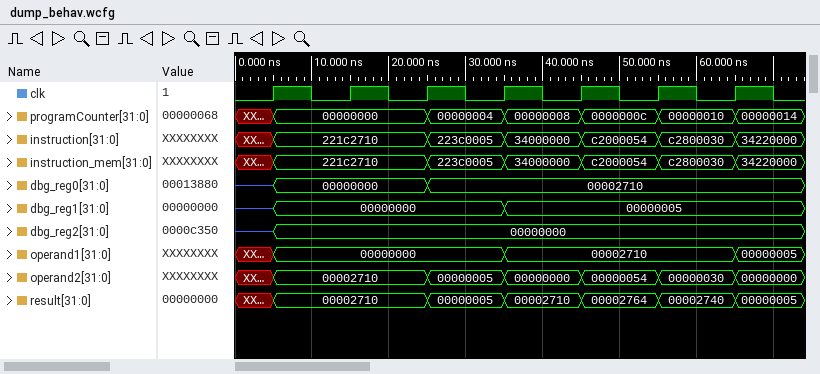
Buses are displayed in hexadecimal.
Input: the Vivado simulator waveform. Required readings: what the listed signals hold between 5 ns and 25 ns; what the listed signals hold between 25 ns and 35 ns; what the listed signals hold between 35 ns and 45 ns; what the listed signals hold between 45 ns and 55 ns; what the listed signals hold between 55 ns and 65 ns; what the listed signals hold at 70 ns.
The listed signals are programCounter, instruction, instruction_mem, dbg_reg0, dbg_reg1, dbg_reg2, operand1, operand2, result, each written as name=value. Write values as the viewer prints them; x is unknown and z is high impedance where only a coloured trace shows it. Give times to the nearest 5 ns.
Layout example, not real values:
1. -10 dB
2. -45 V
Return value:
1. programCounter=00000000, instruction=221c2710, instruction_mem=221c2710, dbg_reg0=00000000, dbg_reg1=00000000, dbg_reg2=00000000, operand1=00000000, operand2=00002710, result=00002710
2. programCounter=00000004, instruction=223c0005, instruction_mem=223c0005, dbg_reg0=00002710, dbg_reg1=00000000, dbg_reg2=00000000, operand1=00000000, operand2=00000005, result=00000005
3. programCounter=00000008, instruction=34000000, instruction_mem=34000000, dbg_reg0=00002710, dbg_reg1=00000005, dbg_reg2=00000000, operand1=00002710, operand2=00000000, result=00002710
4. programCounter=0000000c, instruction=c2000054, instruction_mem=c2000054, dbg_reg0=00002710, dbg_reg1=00000005, dbg_reg2=00000000, operand1=00002710, operand2=00000054, result=00002764
5. programCounter=00000010, instruction=c2800030, instruction_mem=c2800030, dbg_reg0=00002710, dbg_reg1=00000005, dbg_reg2=00000000, operand1=00002710, operand2=00000030, result=00002740
6. programCounter=00000014, instruction=34220000, instruction_mem=34220000, dbg_reg0=00002710, dbg_reg1=00000005, dbg_reg2=00000000, operand1=00000005, operand2=00000000, result=00000005
